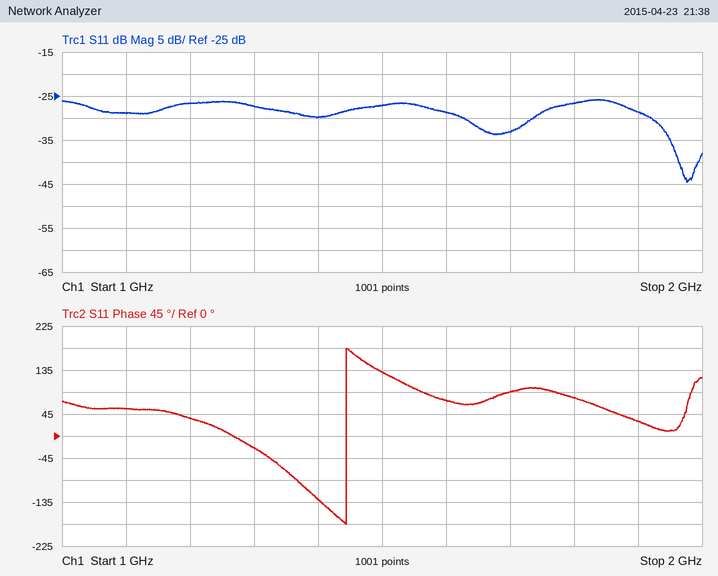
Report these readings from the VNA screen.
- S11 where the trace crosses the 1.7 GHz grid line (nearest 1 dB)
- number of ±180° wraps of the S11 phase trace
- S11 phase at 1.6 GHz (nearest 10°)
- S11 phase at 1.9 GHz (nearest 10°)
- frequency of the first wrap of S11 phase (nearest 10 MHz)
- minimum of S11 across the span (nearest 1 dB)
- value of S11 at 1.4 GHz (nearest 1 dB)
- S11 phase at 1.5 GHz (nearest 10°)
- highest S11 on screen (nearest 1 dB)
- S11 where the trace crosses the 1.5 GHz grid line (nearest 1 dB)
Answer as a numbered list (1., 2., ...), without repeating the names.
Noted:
1. -33 dB
2. 1
3. 70°
4. 30°
5. 1.44 GHz
6. -45 dB
7. -30 dB
8. 130°
9. -26 dB
10. -27 dB
